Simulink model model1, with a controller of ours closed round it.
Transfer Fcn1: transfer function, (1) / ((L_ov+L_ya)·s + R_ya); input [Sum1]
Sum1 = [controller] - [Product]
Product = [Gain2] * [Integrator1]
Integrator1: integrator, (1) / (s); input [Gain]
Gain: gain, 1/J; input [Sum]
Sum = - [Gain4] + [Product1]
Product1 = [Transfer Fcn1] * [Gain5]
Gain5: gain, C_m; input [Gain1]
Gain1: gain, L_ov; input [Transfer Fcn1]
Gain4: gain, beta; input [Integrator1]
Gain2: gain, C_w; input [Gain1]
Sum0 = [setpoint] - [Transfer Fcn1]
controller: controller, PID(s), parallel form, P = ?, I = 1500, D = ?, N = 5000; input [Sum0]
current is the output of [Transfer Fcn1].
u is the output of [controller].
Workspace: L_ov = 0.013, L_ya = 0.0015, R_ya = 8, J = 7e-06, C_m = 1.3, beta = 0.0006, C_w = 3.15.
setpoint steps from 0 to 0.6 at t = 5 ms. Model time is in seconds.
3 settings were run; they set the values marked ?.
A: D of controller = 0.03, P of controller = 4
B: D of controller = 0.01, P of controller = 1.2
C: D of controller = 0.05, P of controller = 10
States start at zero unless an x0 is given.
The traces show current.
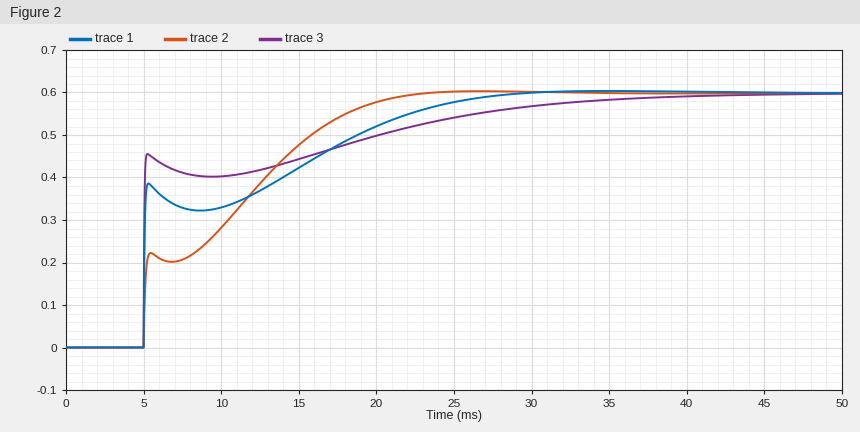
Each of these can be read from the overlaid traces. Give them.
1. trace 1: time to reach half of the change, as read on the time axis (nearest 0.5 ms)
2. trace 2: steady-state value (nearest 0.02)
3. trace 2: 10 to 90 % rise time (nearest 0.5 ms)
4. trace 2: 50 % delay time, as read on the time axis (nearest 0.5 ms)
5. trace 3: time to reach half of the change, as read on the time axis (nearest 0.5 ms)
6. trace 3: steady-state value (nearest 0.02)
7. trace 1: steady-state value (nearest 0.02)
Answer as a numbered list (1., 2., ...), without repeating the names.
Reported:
1. 5.0 ms
2. 0.60
3. 12.5 ms
4. 10.5 ms
5. 5.0 ms
6. 0.60
7. 0.60
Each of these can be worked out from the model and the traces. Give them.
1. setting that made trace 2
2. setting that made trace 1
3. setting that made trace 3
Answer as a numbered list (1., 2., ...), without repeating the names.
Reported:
1. B
2. A
3. C
